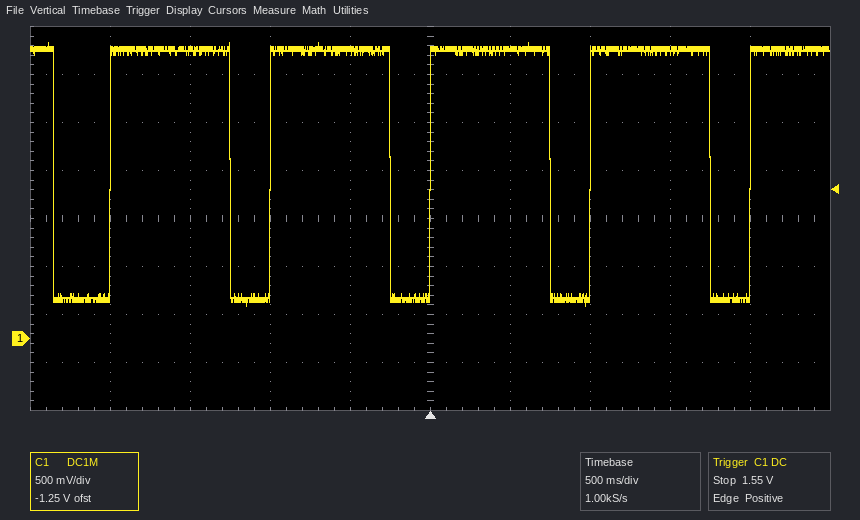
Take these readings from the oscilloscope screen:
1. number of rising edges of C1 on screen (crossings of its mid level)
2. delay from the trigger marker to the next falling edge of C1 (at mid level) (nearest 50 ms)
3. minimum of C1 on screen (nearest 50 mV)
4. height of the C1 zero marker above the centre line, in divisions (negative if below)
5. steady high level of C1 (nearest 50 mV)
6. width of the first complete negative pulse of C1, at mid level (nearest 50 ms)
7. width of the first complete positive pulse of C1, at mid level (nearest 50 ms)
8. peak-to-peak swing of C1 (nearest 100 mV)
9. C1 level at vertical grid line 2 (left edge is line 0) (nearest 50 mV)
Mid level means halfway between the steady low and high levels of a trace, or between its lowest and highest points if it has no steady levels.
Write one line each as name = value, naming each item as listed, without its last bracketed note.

number of rising edges of C1 on screen = 5
delay from the trigger marker to the next falling edge of C1 (at mid level) = 750 ms
minimum of C1 on screen = 350 mV
height of the C1 zero marker above the centre line, in divisions = -2.5 div
steady high level of C1 = 3.00 V
width of the first complete negative pulse of C1, at mid level = 350 ms
width of the first complete positive pulse of C1, at mid level = 750 ms
peak-to-peak swing of C1 = 2.70 V
C1 level at vertical grid line 2 (left edge is line 0) = 3.00 V
